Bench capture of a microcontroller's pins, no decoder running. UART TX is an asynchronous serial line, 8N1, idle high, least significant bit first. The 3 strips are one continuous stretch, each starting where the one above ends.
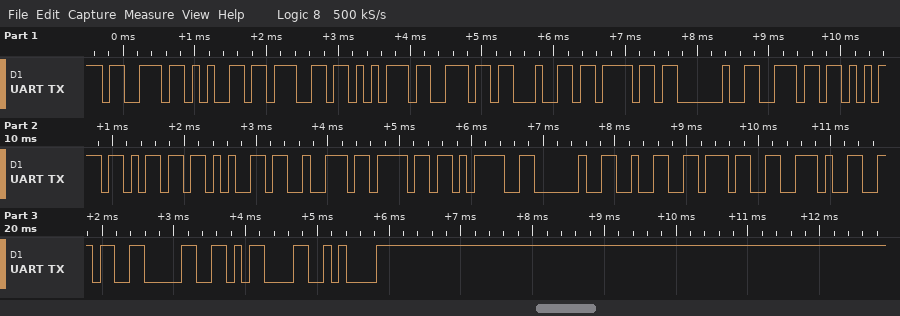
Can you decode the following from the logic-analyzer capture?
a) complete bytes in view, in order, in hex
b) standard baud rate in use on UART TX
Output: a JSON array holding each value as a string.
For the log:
["73 65 67 75 6E 64 6F 20 6E 75 6D 65 72 6F 3D 20 32 37 2E 36 30 0D 0A", "9600 baud"]
